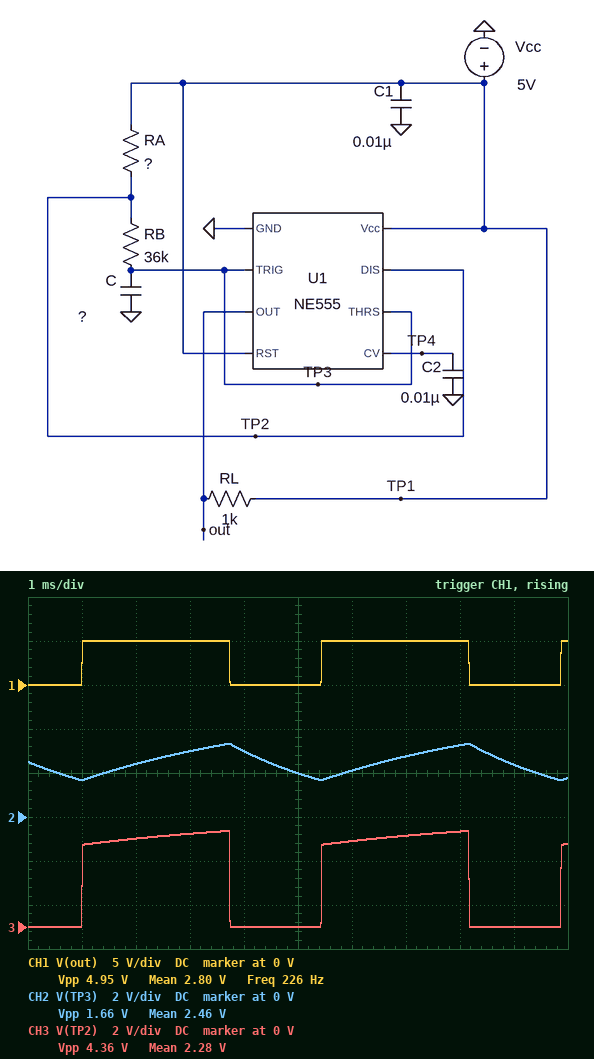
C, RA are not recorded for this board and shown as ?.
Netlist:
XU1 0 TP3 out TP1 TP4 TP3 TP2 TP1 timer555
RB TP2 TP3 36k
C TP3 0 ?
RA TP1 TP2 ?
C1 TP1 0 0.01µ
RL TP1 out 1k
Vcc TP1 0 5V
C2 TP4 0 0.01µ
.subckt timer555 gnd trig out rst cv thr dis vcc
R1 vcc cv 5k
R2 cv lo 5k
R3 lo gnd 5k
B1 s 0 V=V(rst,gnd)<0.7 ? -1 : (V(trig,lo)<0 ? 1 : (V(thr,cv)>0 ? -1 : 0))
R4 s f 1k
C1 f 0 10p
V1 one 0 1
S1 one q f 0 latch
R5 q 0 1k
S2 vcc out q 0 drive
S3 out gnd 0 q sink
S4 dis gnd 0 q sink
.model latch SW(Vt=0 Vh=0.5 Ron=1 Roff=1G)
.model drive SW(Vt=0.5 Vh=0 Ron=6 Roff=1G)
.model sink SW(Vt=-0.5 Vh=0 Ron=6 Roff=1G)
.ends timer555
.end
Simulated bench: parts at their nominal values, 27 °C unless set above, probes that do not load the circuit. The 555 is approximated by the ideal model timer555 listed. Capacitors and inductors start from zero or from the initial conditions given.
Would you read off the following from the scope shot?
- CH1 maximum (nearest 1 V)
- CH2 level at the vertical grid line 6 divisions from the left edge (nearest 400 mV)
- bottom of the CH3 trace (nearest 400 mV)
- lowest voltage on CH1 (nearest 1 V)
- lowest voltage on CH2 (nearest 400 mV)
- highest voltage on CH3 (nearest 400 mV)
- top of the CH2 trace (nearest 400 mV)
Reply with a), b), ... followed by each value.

a) 5 V
b) 2.0 V
c) 0 V
d) 0 V
e) 1.6 V
f) 4.4 V
g) 3.2 V
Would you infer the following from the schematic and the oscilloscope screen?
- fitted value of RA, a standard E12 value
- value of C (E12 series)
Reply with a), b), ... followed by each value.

a) 22 kΩ
b) 68 nF
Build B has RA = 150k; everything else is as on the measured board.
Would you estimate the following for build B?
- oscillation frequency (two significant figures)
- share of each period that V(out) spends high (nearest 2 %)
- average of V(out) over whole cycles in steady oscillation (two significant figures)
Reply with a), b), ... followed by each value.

a) 96 Hz
b) 84 %
c) 4.2 V
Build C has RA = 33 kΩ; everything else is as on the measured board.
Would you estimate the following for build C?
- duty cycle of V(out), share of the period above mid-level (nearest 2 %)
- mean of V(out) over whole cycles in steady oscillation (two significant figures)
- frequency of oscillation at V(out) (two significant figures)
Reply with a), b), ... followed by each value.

a) 66 %
b) 3.3 V
c) 200 Hz
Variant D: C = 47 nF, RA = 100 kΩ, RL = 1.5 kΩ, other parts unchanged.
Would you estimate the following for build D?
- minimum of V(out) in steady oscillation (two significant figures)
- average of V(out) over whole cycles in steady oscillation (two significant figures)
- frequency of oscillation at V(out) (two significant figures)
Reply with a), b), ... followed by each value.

a) 20 mV
b) 4.0 V
c) 180 Hz
